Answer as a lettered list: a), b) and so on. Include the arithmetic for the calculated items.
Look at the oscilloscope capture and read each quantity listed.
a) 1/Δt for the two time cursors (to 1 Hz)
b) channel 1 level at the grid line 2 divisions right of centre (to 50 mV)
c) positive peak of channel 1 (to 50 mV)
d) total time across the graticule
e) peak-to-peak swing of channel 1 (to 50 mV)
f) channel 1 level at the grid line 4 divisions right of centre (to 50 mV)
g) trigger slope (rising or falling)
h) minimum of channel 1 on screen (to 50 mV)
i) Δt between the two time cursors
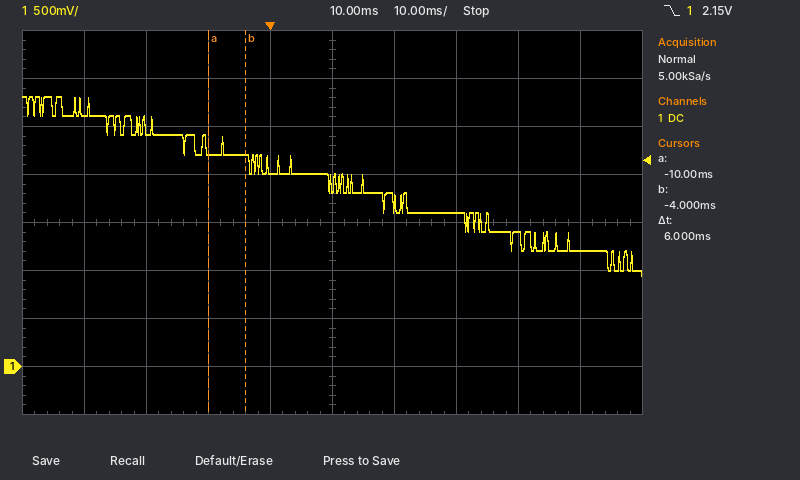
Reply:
a) 1 / 6 ms ≈ 167 Hz
b) 1.60 V
c) 2.80 V
d) 100 ms
e) 2.80 V − (950 mV) = 1.85 V
f) 1.20 V
g) falling
h) 950 mV
i) 6 ms
